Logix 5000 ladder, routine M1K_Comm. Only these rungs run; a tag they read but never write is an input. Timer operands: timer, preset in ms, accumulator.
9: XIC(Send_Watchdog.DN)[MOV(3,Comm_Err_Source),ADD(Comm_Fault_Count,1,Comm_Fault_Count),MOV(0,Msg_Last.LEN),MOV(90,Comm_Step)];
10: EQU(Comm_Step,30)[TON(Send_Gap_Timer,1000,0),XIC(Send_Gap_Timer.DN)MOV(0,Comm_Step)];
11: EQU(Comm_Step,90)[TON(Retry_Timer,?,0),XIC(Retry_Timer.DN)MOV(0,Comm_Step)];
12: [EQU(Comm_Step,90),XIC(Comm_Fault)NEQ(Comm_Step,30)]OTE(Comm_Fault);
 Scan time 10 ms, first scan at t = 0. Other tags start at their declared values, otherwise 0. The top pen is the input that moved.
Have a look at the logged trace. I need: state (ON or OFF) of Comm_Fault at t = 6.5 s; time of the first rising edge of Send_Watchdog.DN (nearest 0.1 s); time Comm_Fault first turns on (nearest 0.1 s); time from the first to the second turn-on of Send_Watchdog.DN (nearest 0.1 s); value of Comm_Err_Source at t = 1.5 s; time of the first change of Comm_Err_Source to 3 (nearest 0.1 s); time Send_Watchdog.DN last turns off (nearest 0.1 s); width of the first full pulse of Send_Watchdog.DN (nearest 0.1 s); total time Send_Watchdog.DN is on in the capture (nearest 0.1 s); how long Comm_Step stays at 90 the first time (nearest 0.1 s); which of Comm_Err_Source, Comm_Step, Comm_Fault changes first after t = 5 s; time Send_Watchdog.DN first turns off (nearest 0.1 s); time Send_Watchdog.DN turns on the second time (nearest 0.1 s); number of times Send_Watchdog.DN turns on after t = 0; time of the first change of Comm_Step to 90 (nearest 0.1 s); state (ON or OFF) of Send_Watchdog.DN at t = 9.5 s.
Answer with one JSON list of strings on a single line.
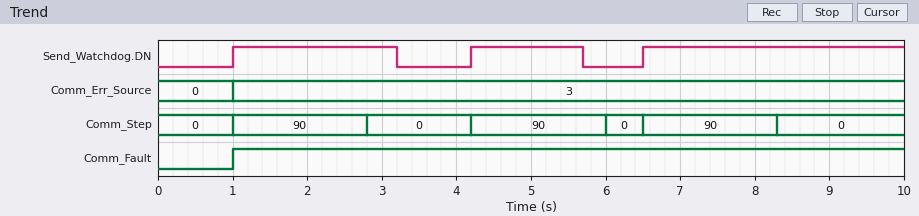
["ON", "1.0 s", "1.0 s", "3.2 s", "3", "1.0 s", "5.7 s", "2.2 s", "7.2 s", "1.8 s", "Comm_Step", "3.2 s", "4.2 s", "3", "1.0 s", "ON"]
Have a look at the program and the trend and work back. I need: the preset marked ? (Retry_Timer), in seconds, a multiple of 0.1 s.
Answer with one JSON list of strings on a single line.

["1.8 s"]
